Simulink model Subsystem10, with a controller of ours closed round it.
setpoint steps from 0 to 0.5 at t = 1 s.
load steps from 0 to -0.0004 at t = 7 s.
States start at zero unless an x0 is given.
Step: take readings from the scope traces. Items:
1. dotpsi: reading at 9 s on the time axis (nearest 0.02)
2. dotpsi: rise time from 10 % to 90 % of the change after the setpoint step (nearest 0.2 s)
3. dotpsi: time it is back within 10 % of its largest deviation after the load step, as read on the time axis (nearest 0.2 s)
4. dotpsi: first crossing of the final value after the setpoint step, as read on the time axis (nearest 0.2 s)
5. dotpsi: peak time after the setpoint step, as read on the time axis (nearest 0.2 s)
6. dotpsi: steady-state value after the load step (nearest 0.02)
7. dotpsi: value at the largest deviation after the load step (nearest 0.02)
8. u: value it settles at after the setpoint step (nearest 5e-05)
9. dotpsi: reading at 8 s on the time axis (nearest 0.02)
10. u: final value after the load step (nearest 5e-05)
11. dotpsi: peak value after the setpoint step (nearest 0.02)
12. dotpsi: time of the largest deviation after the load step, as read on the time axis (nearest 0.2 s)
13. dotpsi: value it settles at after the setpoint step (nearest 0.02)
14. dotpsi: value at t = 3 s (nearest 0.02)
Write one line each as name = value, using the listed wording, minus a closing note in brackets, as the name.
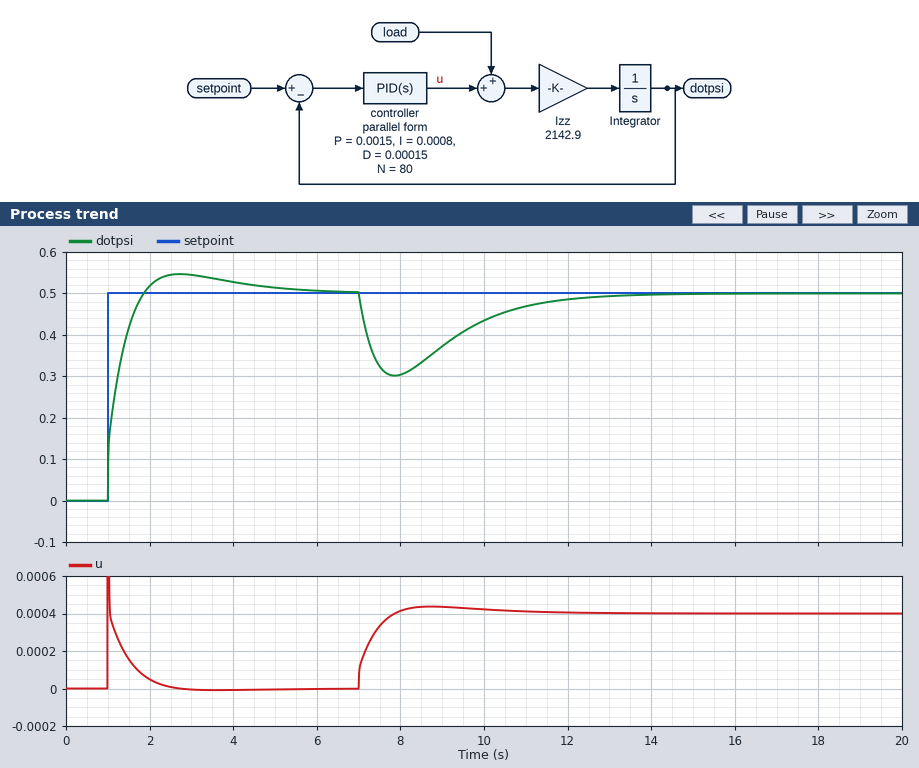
dotpsi: reading at 9 s on the time axis = 0.38
dotpsi: rise time from 10 % to 90 % of the change after the setpoint step = 0.6 s
dotpsi: time it is back within 10 % of its largest deviation after the load step, as read on the time axis = 11.6 s
dotpsi: first crossing of the final value after the setpoint step, as read on the time axis = 1.8 s
dotpsi: peak time after the setpoint step, as read on the time axis = 2.8 s
dotpsi: steady-state value after the load step = 0.50
dotpsi: value at the largest deviation after the load step = 0.30
u: value it settles at after the setpoint step = 0.00000
dotpsi: reading at 8 s on the time axis = 0.30
u: final value after the load step = 0.00040
dotpsi: peak value after the setpoint step = 0.54
dotpsi: time of the largest deviation after the load step, as read on the time axis = 7.8 s
dotpsi: value it settles at after the setpoint step = 0.50
dotpsi: value at t = 3 s = 0.54
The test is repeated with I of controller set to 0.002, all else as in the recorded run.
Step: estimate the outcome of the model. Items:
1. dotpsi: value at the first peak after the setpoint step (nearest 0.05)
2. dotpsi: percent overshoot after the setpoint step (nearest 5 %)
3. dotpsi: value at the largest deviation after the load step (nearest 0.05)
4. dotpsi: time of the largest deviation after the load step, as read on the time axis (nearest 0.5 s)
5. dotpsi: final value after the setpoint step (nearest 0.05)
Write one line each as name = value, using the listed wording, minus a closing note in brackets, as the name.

dotpsi: value at the first peak after the setpoint step = 0.60
dotpsi: percent overshoot after the setpoint step = 15 %
dotpsi: value at the largest deviation after the load step = 0.35
dotpsi: time of the largest deviation after the load step, as read on the time axis = 7.5 s
dotpsi: final value after the setpoint step = 0.50
